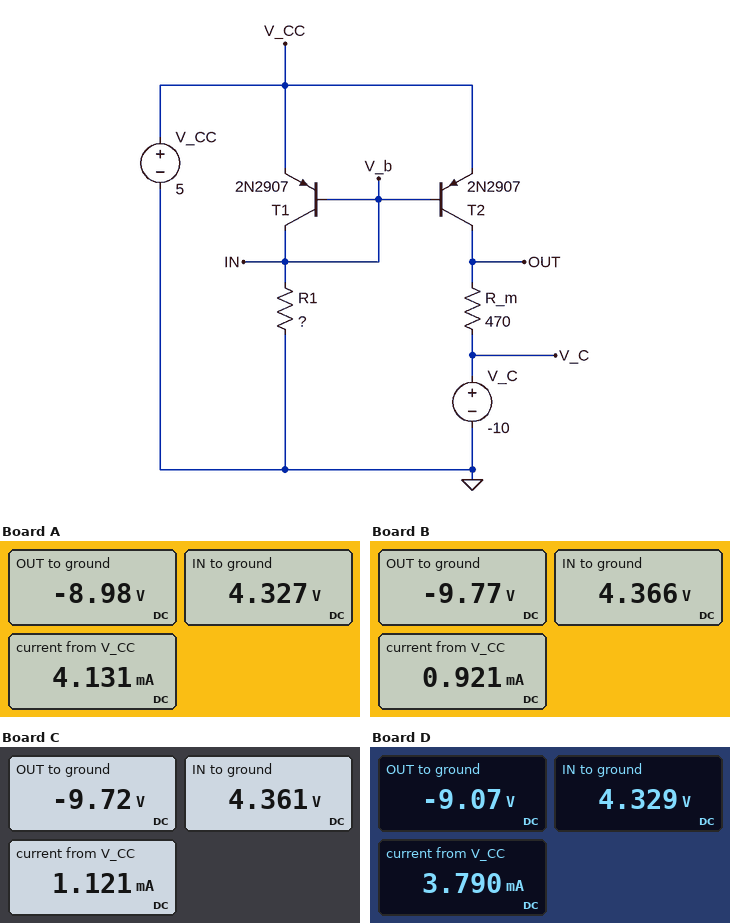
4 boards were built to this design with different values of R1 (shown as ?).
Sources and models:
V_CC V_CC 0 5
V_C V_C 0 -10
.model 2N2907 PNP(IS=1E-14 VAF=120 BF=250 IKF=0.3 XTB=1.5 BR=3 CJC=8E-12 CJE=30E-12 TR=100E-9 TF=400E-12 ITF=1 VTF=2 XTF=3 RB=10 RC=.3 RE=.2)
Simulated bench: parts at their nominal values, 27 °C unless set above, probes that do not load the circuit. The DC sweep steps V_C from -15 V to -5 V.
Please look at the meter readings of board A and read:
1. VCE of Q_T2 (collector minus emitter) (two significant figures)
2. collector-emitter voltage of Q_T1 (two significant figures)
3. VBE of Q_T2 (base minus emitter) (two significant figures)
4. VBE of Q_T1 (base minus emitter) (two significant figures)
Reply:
-14 V
-670 mV
-670 mV
-670 mV
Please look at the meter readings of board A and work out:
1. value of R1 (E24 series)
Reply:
2.2 kΩ
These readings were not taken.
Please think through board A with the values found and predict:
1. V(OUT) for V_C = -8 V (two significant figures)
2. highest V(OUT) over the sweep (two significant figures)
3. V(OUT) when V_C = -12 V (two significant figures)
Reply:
-7.0 V
-4.0 V
-11 V
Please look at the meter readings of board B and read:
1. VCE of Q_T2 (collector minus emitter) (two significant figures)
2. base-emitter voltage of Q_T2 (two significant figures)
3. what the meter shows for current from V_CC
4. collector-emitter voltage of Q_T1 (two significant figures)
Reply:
-15 V
-630 mV
0.921 mA
-630 mV
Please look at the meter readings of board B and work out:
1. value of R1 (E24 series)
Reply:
10 kΩ
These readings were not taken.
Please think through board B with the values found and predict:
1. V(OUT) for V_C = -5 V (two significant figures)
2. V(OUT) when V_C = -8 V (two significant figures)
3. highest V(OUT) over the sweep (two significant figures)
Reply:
-4.8 V
-7.8 V
-4.8 V
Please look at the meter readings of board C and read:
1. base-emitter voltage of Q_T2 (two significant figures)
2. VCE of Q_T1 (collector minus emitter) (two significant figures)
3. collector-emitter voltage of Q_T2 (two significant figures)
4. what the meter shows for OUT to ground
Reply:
-640 mV
-640 mV
-15 V
-9.72 V
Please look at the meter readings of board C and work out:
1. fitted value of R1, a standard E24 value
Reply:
8.2 kΩ
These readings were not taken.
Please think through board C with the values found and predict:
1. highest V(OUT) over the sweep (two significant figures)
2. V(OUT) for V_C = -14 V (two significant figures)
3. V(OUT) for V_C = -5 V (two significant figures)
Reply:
-4.7 V
-14 V
-4.7 V
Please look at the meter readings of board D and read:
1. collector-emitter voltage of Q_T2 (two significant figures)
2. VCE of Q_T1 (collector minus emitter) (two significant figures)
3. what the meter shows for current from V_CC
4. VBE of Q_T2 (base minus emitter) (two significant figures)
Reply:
-14 V
-670 mV
3.790 mA
-670 mV
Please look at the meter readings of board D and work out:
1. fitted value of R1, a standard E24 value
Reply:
2.4 kΩ
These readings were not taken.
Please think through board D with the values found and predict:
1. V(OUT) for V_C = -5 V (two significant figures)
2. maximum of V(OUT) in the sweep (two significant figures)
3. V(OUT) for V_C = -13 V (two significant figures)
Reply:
-4.1 V
-4.1 V
-12 V
